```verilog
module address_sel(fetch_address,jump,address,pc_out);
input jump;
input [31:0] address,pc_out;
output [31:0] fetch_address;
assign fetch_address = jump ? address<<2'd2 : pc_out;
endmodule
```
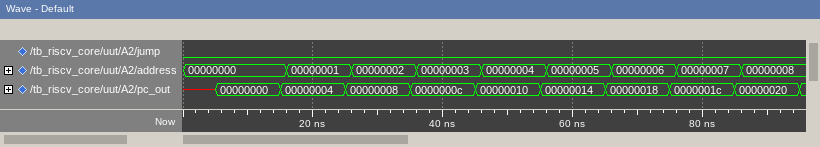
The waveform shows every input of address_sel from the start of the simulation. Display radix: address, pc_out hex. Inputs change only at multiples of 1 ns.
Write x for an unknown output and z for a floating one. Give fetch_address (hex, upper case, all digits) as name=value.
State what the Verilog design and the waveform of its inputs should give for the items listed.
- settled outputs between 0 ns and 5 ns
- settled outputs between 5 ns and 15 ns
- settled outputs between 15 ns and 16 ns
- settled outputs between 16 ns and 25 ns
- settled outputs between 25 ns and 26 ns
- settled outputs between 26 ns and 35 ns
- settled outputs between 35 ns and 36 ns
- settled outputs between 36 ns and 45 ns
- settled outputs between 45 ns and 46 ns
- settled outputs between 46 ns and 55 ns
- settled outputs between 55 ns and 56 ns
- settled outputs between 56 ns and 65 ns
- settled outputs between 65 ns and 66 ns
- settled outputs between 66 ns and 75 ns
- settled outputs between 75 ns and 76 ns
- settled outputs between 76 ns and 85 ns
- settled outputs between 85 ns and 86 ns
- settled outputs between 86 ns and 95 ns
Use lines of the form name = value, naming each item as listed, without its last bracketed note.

settled outputs between 0 ns and 5 ns = fetch_address=x
settled outputs between 5 ns and 15 ns = fetch_address=00000000
settled outputs between 15 ns and 16 ns = fetch_address=00000004
settled outputs between 16 ns and 25 ns = fetch_address=00000004
settled outputs between 25 ns and 26 ns = fetch_address=00000008
settled outputs between 26 ns and 35 ns = fetch_address=00000008
settled outputs between 35 ns and 36 ns = fetch_address=0000000C
settled outputs between 36 ns and 45 ns = fetch_address=0000000C
settled outputs between 45 ns and 46 ns = fetch_address=00000010
settled outputs between 46 ns and 55 ns = fetch_address=00000010
settled outputs between 55 ns and 56 ns = fetch_address=00000014
settled outputs between 56 ns and 65 ns = fetch_address=00000014
settled outputs between 65 ns and 66 ns = fetch_address=00000018
settled outputs between 66 ns and 75 ns = fetch_address=00000018
settled outputs between 75 ns and 76 ns = fetch_address=0000001C
settled outputs between 76 ns and 85 ns = fetch_address=0000001C
settled outputs between 85 ns and 86 ns = fetch_address=00000020
settled outputs between 86 ns and 95 ns = fetch_address=00000020
